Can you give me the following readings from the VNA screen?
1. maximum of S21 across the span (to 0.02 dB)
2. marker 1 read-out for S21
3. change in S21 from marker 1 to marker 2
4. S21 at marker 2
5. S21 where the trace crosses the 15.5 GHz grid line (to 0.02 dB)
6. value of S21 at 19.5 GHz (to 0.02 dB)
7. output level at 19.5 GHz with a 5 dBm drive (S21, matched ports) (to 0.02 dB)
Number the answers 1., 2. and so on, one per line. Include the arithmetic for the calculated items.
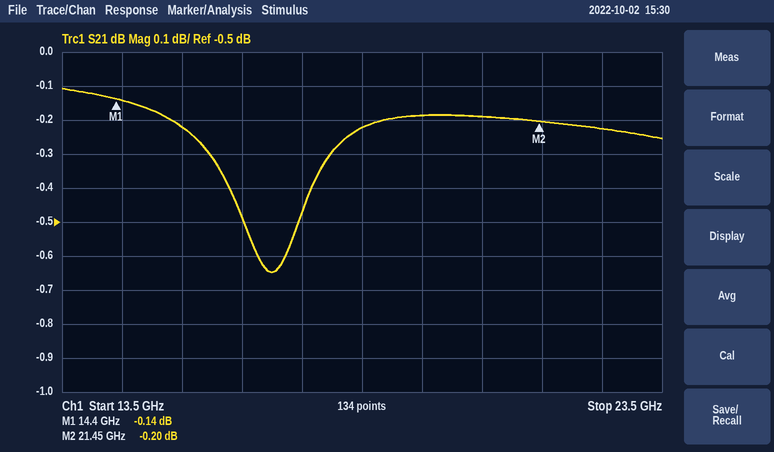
1. -0.10 dB
2. -0.14 dB
3. -0.2 − (-0.14) = -0.06 dB
4. -0.20 dB
5. -0.22 dB
6. -0.18 dB
7. 5 dBm + (-0.18 dB) = 4.82 dBm
